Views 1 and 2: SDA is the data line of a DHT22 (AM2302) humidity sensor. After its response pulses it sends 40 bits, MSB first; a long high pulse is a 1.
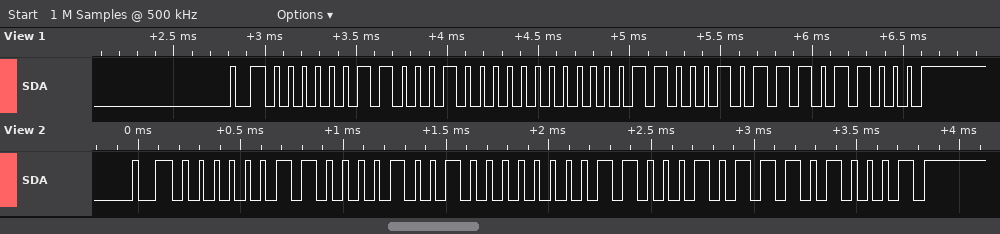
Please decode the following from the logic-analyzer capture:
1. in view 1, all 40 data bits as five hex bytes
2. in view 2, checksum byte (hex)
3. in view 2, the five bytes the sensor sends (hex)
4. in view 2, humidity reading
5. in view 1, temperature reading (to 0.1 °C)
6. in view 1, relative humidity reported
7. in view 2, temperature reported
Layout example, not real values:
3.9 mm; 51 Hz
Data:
03 10 00 C5 D8; 0xD1; 03 09 00 C5 D1; 77.7 %; 19.7 °C; 78.4 %; 19.7 °C
